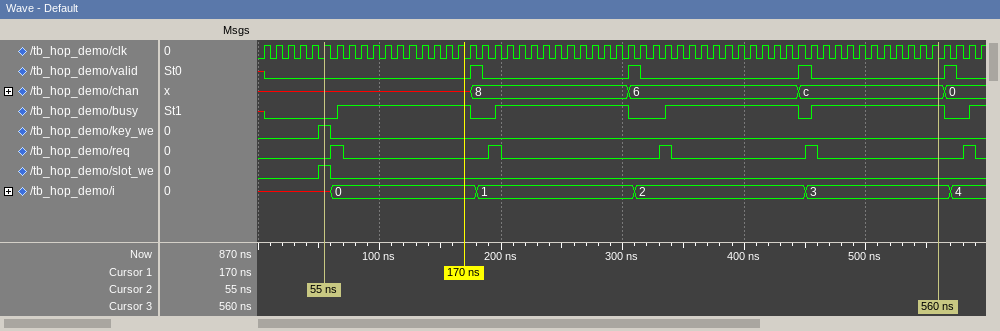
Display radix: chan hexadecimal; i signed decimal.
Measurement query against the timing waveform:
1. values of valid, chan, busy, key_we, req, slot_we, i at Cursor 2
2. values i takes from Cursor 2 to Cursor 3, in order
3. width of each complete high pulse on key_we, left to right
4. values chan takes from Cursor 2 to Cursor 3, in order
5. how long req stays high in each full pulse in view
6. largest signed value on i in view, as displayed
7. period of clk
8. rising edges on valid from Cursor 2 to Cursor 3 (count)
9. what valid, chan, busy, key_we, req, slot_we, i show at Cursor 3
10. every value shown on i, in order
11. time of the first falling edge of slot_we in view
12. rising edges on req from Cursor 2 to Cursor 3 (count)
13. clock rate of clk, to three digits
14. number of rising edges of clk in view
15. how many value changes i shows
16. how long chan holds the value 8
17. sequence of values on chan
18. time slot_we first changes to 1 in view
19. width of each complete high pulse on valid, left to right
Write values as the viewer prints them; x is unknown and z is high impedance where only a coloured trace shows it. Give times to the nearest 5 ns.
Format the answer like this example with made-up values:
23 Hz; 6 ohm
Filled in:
valid=0, chan=x, busy=0, key_we=1, req=0, slot_we=1, i=x; x, 0, 1, 2, 3; 10 ns; x, 8, 6, c; 10 ns, 10 ns, 10 ns, 10 ns, 10 ns; 4; 10 ns; 3; valid=0, chan=c, busy=1, key_we=0, req=0, slot_we=0, i=3; x, 0, 1, 2, 3, 4; 60 ns; 4; 100 MHz; 60; 5; 130 ns; x, 8, 6, c, 0; 50 ns; 10 ns, 10 ns, 10 ns, 10 ns
